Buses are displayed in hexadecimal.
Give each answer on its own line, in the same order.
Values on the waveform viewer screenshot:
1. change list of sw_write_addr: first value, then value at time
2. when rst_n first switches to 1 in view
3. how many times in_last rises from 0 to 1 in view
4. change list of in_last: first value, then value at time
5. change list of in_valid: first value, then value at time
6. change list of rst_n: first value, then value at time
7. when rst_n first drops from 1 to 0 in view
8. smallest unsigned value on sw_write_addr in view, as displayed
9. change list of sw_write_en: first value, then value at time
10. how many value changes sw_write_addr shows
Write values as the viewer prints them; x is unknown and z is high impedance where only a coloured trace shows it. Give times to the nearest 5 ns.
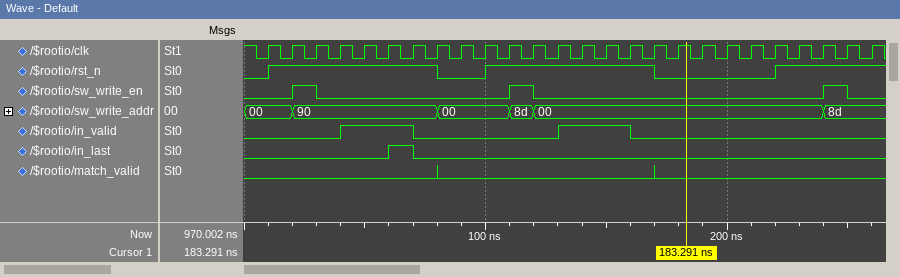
00, 90 at 20 ns, 00 at 80 ns, 8d at 110 ns, 00 at 120 ns, 8d at 240 ns
10 ns
1
0, 1 at 60 ns, 0 at 70 ns
0, 1 at 40 ns, 0 at 70 ns, 1 at 130 ns, 0 at 160 ns
0, 1 at 10 ns, 0 at 80 ns, 1 at 100 ns, 0 at 170 ns, 1 at 220 ns
80 ns
00
0, 1 at 20 ns, 0 at 30 ns, 1 at 110 ns, 0 at 120 ns, 1 at 240 ns, 0 at 250 ns
5
